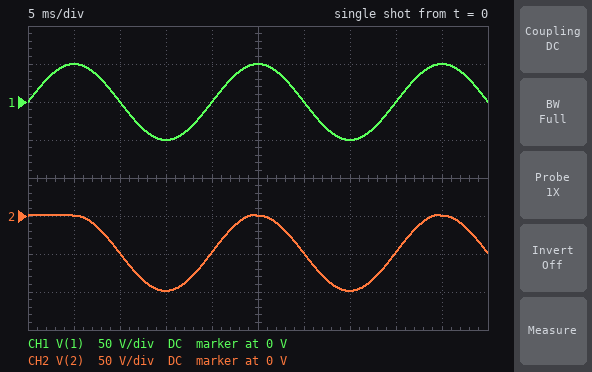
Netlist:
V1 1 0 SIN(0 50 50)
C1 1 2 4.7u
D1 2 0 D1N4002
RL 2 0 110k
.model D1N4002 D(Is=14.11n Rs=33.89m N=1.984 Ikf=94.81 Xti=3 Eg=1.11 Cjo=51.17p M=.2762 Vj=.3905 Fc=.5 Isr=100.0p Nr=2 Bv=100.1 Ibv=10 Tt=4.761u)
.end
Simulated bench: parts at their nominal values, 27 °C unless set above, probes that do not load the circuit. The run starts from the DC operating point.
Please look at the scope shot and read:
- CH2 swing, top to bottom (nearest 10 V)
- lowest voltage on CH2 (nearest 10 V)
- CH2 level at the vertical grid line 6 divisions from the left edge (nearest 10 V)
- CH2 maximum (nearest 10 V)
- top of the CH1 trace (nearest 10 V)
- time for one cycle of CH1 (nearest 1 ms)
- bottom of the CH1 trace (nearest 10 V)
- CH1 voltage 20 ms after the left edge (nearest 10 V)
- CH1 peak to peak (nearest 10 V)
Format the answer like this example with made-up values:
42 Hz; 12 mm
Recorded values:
100 V; -100 V; -50 V; 0 V; 50 V; 20 ms; -50 V; 0 V; 100 V
